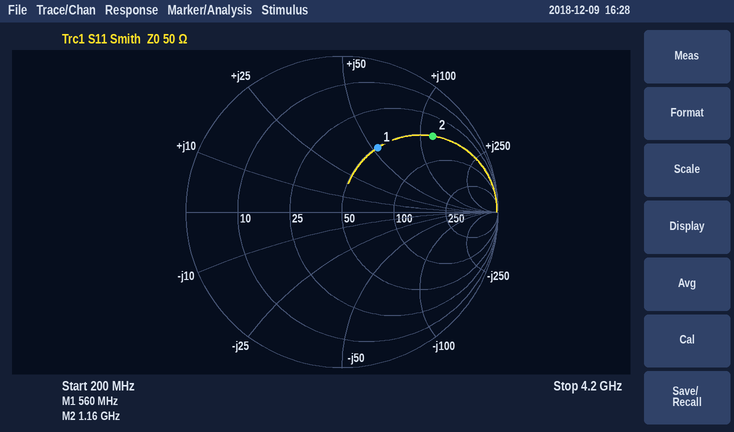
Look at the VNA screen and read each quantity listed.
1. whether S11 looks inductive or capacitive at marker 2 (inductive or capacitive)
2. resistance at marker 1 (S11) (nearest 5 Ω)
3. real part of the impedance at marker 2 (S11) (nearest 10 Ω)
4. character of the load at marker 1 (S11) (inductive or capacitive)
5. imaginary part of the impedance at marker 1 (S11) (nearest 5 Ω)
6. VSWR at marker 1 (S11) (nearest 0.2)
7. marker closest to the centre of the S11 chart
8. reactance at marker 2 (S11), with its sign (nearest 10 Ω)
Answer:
inductive
50 Ω
50 Ω
inductive
+55 Ω
2.8
marker 1
+120 Ω
